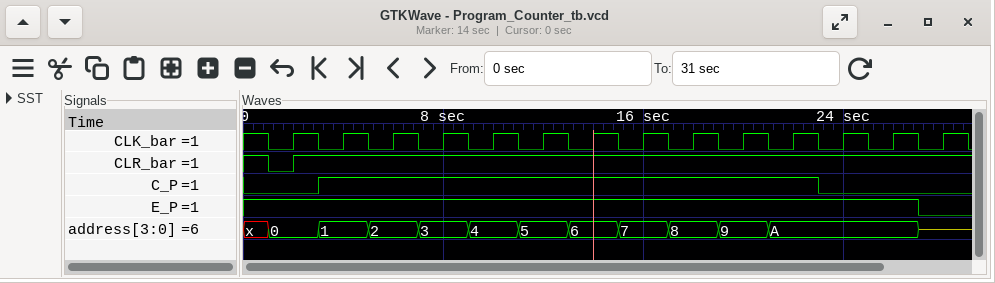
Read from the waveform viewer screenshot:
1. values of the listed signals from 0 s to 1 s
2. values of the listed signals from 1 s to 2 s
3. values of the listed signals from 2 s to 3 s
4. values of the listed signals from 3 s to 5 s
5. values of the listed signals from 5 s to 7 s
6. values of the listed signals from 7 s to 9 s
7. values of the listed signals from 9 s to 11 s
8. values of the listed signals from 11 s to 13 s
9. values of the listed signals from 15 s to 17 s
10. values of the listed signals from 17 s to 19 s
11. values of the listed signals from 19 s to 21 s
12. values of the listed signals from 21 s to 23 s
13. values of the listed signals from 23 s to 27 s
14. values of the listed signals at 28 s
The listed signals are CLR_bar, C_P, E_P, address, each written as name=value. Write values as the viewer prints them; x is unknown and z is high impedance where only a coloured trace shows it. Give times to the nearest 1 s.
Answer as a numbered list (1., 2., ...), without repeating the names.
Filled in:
1. CLR_bar=1, C_P=0, E_P=1, address=x
2. CLR_bar=0, C_P=0, E_P=1, address=0
3. CLR_bar=1, C_P=0, E_P=1, address=0
4. CLR_bar=1, C_P=1, E_P=1, address=1
5. CLR_bar=1, C_P=1, E_P=1, address=2
6. CLR_bar=1, C_P=1, E_P=1, address=3
7. CLR_bar=1, C_P=1, E_P=1, address=4
8. CLR_bar=1, C_P=1, E_P=1, address=5
9. CLR_bar=1, C_P=1, E_P=1, address=7
10. CLR_bar=1, C_P=1, E_P=1, address=8
11. CLR_bar=1, C_P=1, E_P=1, address=9
12. CLR_bar=1, C_P=1, E_P=1, address=A
13. CLR_bar=1, C_P=0, E_P=1, address=A
14. CLR_bar=1, C_P=0, E_P=0, address=z
